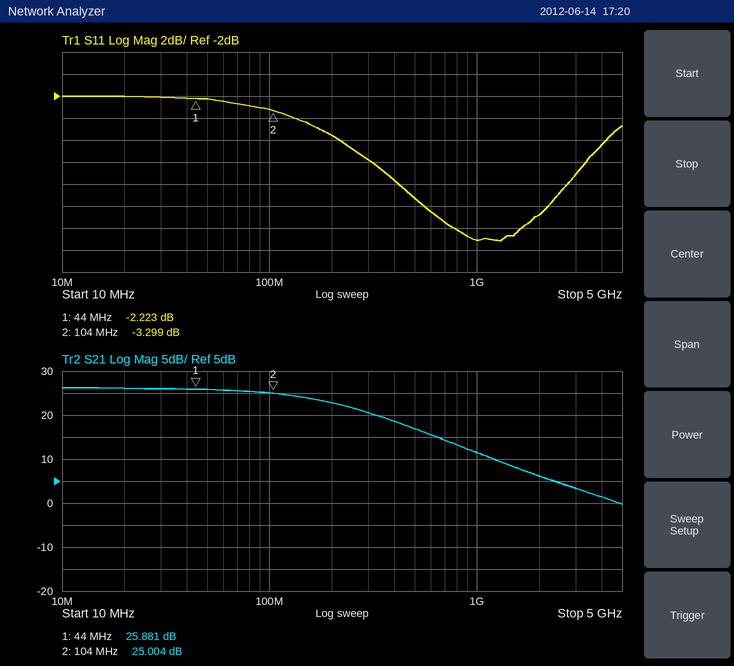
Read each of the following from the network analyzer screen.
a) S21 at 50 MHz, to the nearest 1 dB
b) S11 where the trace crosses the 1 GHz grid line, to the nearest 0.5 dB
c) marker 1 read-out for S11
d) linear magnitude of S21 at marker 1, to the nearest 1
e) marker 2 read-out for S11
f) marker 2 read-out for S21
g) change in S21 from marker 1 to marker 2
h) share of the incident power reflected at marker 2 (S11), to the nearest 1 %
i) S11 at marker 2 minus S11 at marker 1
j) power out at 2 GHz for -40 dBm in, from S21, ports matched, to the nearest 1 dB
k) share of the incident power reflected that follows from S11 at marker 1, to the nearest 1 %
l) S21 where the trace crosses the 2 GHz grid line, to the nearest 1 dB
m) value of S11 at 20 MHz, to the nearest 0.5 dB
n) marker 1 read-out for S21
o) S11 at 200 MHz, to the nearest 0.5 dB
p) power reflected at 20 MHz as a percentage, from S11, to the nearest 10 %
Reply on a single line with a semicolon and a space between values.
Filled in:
26 dB; -15.0 dB; -2.223 dB; 20; -3.299 dB; 25.004 dB; -0.877 dB; 47 %; -1.076 dB; -34 dBm; 60 %; 6 dB; -2.0 dB; 25.881 dB; -5.5 dB; 60 %
